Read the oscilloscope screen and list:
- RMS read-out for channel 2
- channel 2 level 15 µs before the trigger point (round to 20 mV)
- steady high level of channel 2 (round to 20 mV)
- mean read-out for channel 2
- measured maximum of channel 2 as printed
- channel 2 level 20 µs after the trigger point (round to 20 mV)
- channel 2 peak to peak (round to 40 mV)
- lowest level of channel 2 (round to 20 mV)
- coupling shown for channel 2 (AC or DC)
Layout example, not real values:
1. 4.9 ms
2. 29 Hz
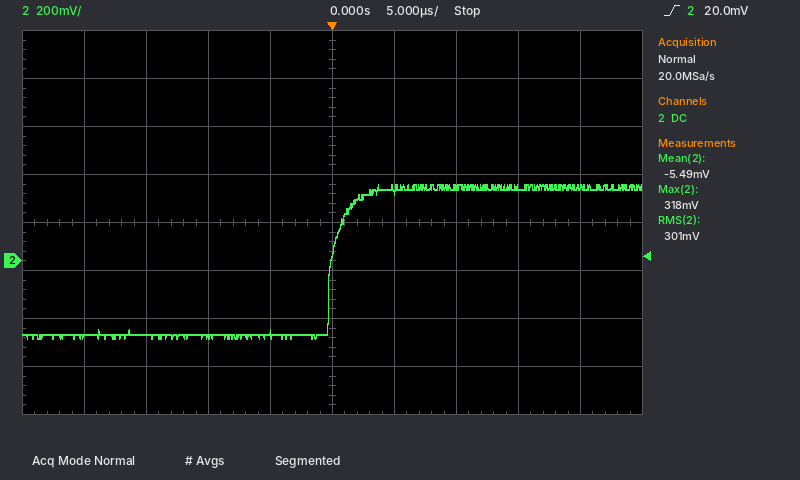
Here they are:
1. 301 mV
2. -300 mV
3. 300 mV
4. -5.49 mV
5. 318 mV
6. 300 mV
7. 640 mV
8. -320 mV
9. DC
